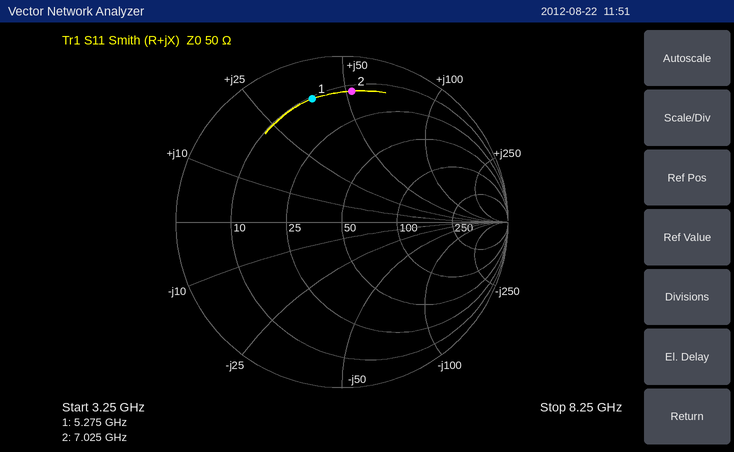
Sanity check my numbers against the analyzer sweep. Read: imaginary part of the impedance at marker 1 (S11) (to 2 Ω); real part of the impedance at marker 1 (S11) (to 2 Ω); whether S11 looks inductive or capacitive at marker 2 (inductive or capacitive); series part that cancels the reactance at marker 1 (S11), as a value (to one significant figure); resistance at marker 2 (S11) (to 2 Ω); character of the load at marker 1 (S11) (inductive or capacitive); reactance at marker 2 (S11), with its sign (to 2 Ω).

+38 Ω
10 Ω
inductive
800 fF
12 Ω
inductive
+52 Ω
